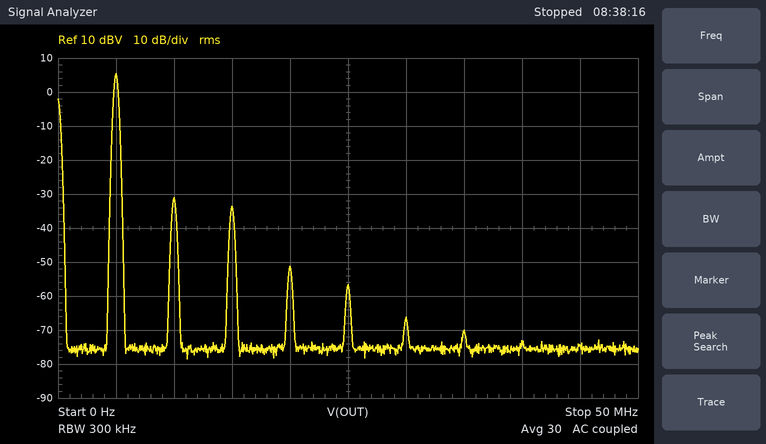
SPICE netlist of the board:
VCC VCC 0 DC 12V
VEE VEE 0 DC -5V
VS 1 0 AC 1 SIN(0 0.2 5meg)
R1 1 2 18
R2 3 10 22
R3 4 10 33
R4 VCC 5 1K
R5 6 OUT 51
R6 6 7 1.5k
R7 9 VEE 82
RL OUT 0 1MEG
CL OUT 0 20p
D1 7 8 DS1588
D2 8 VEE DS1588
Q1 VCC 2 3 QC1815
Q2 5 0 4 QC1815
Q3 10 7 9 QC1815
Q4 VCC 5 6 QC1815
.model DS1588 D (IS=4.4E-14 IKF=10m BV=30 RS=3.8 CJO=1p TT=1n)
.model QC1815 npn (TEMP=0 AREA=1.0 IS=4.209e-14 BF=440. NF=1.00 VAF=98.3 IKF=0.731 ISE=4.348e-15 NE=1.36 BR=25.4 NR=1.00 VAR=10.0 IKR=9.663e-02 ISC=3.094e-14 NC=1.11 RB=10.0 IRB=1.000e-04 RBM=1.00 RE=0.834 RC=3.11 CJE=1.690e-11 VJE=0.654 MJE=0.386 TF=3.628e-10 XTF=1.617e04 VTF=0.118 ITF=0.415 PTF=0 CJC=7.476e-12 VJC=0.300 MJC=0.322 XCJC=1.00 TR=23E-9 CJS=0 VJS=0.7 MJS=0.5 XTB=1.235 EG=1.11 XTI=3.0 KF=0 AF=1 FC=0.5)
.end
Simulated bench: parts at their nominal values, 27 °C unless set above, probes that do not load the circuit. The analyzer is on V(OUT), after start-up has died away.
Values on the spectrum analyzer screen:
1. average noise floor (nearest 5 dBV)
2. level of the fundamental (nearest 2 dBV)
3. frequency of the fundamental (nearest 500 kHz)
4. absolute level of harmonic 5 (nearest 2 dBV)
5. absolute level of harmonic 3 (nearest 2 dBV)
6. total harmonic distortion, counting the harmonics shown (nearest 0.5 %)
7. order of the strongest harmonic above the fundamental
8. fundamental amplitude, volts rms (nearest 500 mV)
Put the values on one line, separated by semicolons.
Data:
-75 dBV; 6 dBV; 5.0 MHz; -56 dBV; -34 dBV; 2.0 %; 2; 2.0 V
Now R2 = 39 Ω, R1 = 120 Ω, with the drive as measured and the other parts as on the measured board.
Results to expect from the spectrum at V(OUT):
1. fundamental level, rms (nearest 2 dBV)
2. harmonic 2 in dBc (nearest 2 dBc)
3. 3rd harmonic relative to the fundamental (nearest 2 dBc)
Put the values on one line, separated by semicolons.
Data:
4 dBV; -42 dBc; -46 dBc
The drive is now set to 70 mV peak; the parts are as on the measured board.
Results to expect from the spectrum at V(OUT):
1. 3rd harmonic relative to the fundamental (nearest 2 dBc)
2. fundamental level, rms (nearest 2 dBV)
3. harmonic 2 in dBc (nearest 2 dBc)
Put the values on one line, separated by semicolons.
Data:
-60 dBc; -4 dBV; -48 dBc
